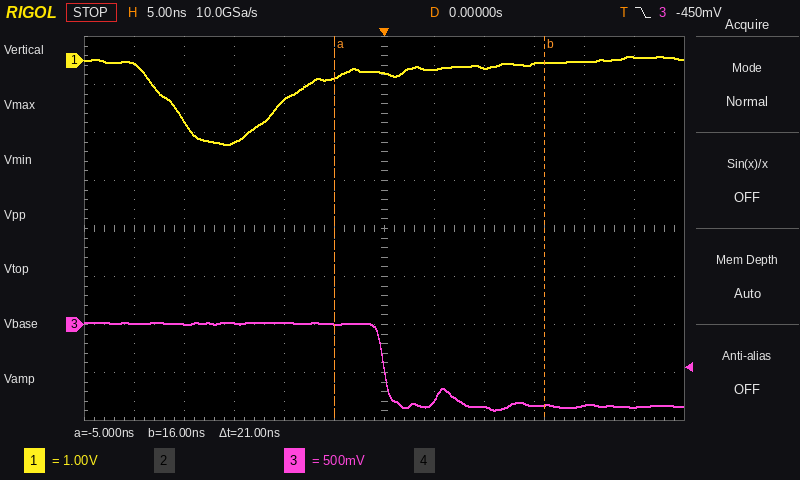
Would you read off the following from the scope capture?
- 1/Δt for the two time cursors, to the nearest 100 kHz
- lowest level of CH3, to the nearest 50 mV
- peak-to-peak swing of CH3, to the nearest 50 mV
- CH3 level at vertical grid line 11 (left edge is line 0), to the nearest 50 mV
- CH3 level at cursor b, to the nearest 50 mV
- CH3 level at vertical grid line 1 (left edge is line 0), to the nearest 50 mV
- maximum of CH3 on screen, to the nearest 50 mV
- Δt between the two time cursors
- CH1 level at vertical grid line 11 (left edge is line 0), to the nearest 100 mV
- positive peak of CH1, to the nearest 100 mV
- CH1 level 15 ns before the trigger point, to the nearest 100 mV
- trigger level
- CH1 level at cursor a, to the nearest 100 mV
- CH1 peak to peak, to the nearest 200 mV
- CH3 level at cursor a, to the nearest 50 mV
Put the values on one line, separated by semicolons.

47.6 MHz; -900 mV; 900 mV; -850 mV; -850 mV; 0 mV; 0 mV; 21 ns; 100 mV; 100 mV; -1.7 V; -450 mV; -400 mV; 1.8 V; 0 mV
